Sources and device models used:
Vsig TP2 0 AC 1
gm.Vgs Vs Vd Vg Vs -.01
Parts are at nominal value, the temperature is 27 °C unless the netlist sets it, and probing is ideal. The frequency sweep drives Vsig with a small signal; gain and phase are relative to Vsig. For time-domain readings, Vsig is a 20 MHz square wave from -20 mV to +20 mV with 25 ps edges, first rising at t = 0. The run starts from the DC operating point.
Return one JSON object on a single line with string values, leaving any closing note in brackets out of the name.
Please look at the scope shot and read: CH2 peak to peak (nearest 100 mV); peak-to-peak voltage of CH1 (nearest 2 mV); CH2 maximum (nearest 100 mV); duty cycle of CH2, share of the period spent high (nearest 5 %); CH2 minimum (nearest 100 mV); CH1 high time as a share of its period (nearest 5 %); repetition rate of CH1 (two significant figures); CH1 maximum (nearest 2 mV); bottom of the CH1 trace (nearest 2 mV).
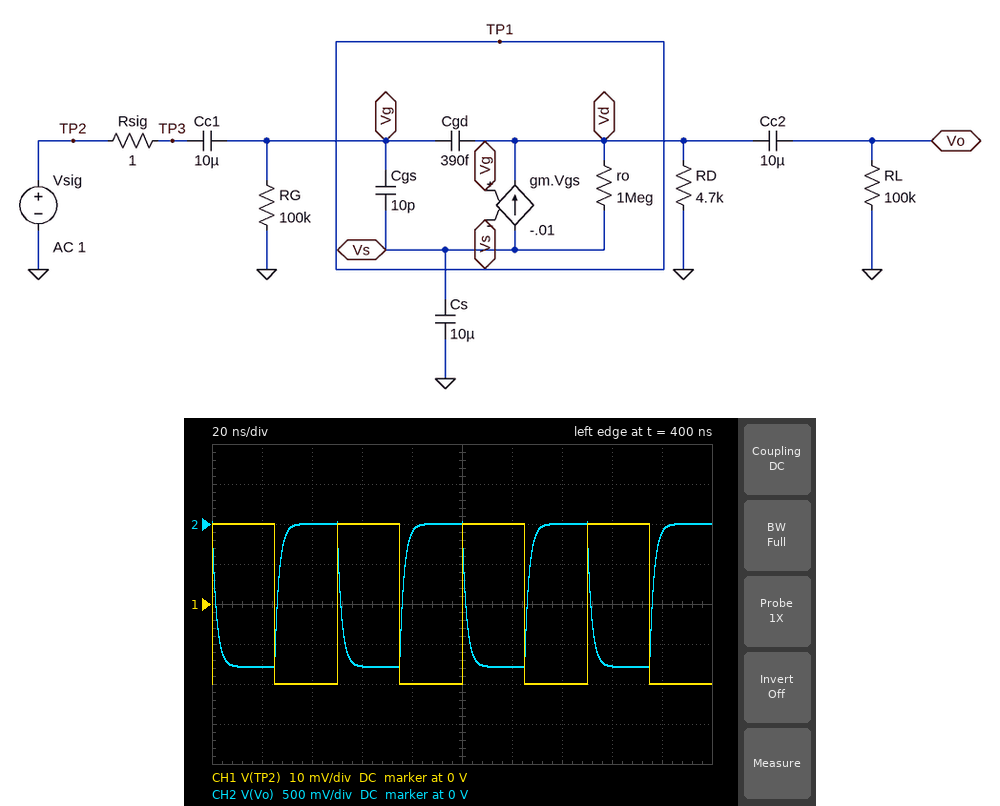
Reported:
{"CH2 peak to peak": "1.8 V", "peak-to-peak voltage of CH1": "40 mV", "CH2 maximum": "0 V", "duty cycle of CH2, share of the period spent high": "50 %", "CH2 minimum": "-1.8 V", "CH1 high time as a share of its period": "50 %", "repetition rate of CH1": "20 MHz", "CH1 maximum": "20 mV", "bottom of the CH1 trace": "-20 mV"}
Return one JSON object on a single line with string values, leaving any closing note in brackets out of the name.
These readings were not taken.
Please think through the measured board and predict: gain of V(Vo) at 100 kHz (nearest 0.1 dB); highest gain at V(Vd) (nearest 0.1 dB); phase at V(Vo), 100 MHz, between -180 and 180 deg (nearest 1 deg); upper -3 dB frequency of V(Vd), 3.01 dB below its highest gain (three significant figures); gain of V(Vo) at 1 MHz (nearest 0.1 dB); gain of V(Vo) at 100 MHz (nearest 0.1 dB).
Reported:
{"gain of V(Vo) at 100 kHz": "33.0 dB", "highest gain at V(Vd)": "33.0 dB", "phase at V(Vo), 100 MHz, between -180 and 180 deg": "130 deg", "upper -3 dB frequency of V(Vd), 3.01 dB below its highest gain": "90.4 MHz", "gain of V(Vo) at 1 MHz": "33.0 dB", "gain of V(Vo) at 100 MHz": "29.5 dB"}
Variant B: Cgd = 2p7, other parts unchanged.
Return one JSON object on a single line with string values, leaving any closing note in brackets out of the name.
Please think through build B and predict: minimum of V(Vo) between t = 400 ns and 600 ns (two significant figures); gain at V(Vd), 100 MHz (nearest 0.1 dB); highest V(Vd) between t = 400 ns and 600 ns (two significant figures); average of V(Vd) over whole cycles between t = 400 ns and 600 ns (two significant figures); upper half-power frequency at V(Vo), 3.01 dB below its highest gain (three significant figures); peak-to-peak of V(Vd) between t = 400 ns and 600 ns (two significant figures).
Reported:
{"minimum of V(Vo) between t = 400 ns and 600 ns": "-1.6 V", "gain at V(Vd), 100 MHz": "15.4 dB", "highest V(Vd) between t = 400 ns and 600 ns": "-170 mV", "average of V(Vd) over whole cycles between t = 400 ns and 600 ns": "-890 mV", "upper half-power frequency at V(Vo), 3.01 dB below its highest gain": "13.1 MHz", "peak-to-peak of V(Vd) between t = 400 ns and 600 ns": "1.4 V"}
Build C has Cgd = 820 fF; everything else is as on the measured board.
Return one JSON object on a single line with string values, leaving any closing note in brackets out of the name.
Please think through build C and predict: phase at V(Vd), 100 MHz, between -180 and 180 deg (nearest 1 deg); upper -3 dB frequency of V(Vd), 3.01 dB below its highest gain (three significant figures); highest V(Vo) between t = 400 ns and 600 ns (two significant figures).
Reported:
{"phase at V(Vd), 100 MHz, between -180 and 180 deg": "110 deg", "upper -3 dB frequency of V(Vd), 3.01 dB below its highest gain": "43.0 MHz", "highest V(Vo) between t = 400 ns and 600 ns": "26 mV"}
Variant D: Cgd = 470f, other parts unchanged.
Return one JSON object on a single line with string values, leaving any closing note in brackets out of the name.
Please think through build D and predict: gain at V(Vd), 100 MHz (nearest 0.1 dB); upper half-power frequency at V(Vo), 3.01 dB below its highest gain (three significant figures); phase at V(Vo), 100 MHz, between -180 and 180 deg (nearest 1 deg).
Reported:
{"gain at V(Vd), 100 MHz": "28.6 dB", "upper half-power frequency at V(Vo), 3.01 dB below its highest gain": "75.0 MHz", "phase at V(Vo), 100 MHz, between -180 and 180 deg": "125 deg"}
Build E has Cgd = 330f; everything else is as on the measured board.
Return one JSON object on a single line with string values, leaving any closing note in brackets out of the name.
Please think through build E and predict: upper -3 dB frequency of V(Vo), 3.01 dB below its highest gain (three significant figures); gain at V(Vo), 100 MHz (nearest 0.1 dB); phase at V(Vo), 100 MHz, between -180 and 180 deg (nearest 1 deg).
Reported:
{"upper -3 dB frequency of V(Vo), 3.01 dB below its highest gain": "107 MHz", "gain at V(Vo), 100 MHz": "30.3 dB", "phase at V(Vo), 100 MHz, between -180 and 180 deg": "135 deg"}
